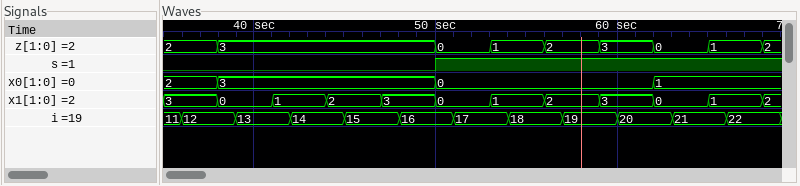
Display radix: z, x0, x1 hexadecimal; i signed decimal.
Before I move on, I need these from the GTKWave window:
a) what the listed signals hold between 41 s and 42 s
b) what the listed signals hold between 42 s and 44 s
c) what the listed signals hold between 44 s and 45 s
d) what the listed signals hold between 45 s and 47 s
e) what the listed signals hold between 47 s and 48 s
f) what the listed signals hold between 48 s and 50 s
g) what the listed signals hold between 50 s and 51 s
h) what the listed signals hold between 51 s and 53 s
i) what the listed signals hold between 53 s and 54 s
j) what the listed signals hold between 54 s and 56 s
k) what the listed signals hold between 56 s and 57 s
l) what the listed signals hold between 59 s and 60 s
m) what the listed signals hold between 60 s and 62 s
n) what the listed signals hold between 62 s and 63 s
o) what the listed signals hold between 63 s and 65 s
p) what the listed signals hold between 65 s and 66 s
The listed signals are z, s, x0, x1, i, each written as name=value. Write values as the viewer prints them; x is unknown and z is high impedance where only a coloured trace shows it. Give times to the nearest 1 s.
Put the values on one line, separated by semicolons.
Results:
z=3, s=0, x0=3, x1=1, i=13; z=3, s=0, x0=3, x1=1, i=14; z=3, s=0, x0=3, x1=2, i=14; z=3, s=0, x0=3, x1=2, i=15; z=3, s=0, x0=3, x1=3, i=15; z=3, s=0, x0=3, x1=3, i=16; z=0, s=1, x0=0, x1=0, i=16; z=0, s=1, x0=0, x1=0, i=17; z=1, s=1, x0=0, x1=1, i=17; z=1, s=1, x0=0, x1=1, i=18; z=2, s=1, x0=0, x1=2, i=18; z=3, s=1, x0=0, x1=3, i=19; z=3, s=1, x0=0, x1=3, i=20; z=0, s=1, x0=1, x1=0, i=20; z=0, s=1, x0=1, x1=0, i=21; z=1, s=1, x0=1, x1=1, i=21
